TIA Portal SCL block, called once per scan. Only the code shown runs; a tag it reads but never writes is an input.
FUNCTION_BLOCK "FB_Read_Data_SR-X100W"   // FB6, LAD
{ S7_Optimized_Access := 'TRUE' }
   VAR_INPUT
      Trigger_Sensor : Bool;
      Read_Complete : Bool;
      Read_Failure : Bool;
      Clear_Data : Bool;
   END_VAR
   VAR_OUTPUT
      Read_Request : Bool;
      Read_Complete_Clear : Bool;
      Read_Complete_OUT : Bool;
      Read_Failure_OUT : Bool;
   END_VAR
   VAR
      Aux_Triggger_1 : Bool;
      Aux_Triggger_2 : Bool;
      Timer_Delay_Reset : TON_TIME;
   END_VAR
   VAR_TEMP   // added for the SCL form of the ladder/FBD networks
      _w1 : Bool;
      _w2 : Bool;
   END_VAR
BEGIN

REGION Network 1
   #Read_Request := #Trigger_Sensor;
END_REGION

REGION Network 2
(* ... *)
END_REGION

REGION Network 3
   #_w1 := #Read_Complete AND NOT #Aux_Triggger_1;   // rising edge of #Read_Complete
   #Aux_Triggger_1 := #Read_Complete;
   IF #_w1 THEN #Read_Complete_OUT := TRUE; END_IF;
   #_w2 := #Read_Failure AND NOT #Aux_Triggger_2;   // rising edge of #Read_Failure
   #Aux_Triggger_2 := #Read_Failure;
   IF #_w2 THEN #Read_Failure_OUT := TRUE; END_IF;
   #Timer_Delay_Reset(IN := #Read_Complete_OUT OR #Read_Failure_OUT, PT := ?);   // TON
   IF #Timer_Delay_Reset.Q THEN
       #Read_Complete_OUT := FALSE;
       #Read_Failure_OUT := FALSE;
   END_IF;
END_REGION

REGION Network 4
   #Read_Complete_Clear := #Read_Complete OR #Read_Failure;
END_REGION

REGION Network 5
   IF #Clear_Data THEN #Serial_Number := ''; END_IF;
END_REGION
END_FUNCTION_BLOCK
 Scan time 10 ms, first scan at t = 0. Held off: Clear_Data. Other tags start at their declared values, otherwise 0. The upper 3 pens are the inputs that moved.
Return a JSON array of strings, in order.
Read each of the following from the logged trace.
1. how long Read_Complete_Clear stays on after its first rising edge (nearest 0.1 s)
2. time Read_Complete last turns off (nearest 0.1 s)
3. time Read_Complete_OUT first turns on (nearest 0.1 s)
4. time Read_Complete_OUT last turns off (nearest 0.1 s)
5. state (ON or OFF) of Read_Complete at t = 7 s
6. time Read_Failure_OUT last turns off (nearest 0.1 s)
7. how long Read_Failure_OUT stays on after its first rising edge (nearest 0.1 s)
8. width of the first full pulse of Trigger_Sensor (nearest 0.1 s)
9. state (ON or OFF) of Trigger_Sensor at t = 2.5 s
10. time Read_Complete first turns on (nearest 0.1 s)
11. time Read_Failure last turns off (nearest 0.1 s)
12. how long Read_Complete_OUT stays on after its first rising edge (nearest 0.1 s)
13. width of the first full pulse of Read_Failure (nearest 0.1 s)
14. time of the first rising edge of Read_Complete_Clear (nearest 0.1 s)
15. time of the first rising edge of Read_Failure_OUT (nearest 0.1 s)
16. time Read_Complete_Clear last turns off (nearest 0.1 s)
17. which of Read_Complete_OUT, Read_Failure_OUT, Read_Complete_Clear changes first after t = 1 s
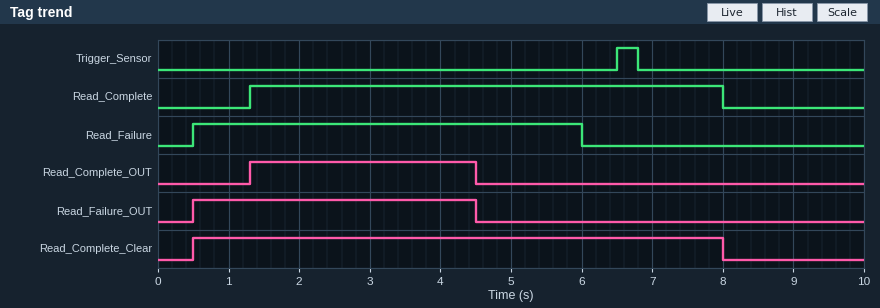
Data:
["7.5 s", "8.0 s", "1.3 s", "4.5 s", "ON", "4.5 s", "4.0 s", "0.3 s", "OFF", "1.3 s", "6.0 s", "3.2 s", "5.5 s", "0.5 s", "0.5 s", "8.0 s", "Read_Complete_OUT"]
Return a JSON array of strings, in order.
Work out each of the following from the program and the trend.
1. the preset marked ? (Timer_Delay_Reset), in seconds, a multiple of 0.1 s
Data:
["4.0 s"]
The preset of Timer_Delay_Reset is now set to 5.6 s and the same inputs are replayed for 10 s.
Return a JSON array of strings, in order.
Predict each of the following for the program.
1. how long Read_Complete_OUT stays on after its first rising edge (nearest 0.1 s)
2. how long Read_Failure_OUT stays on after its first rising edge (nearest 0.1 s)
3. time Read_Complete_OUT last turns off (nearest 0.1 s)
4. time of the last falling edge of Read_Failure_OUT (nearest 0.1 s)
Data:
["4.8 s", "5.6 s", "6.1 s", "6.1 s"]
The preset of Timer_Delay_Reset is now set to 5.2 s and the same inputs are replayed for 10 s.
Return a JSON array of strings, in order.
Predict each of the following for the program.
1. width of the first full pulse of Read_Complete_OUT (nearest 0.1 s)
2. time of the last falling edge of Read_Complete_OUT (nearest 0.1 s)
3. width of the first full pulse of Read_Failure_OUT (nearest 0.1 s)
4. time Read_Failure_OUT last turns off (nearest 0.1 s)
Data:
["4.4 s", "5.7 s", "5.2 s", "5.7 s"]
